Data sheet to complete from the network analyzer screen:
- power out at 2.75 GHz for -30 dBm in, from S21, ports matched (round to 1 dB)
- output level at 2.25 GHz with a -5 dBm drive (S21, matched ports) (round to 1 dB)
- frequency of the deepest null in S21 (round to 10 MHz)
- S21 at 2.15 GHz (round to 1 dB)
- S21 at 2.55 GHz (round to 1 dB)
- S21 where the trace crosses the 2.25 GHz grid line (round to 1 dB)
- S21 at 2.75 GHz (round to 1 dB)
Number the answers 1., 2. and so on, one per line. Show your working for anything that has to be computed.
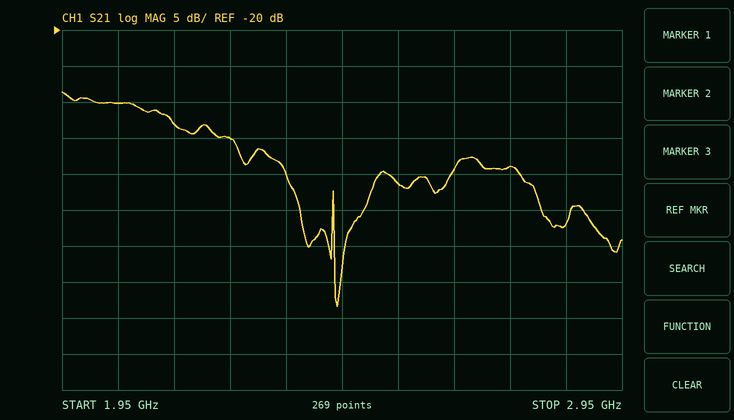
1. -30 dBm + (-39 dB) = -69 dBm
2. -5 dBm + (-35 dB) = -40 dBm
3. 2.44 GHz
4. -33 dB
5. -41 dB
6. -35 dB
7. -39 dB
